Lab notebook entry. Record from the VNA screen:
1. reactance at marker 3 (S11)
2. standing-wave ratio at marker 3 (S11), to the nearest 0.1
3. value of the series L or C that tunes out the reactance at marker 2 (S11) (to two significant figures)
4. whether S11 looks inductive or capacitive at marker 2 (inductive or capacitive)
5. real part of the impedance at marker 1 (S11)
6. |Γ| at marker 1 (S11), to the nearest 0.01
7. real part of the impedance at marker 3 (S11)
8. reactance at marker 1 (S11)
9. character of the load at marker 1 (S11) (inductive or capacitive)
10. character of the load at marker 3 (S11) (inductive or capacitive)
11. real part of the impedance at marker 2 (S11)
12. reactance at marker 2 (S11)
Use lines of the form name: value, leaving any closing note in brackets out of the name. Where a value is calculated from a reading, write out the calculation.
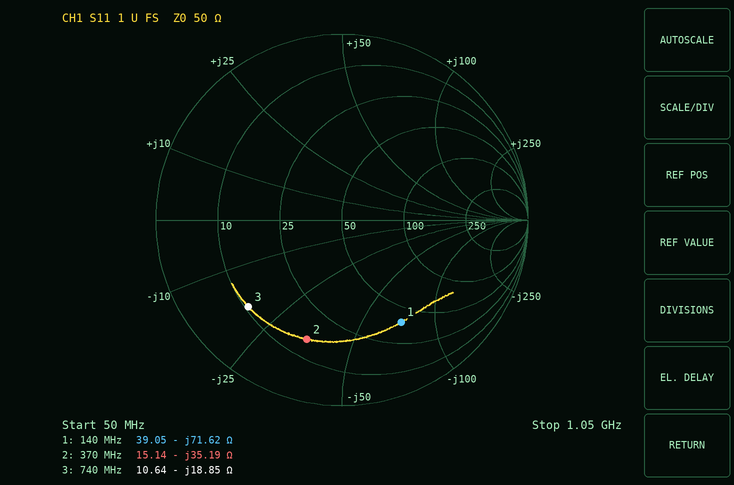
reactance at marker 3: -18.85 Ω
standing-wave ratio at marker 3 (S11), to the nearest 0.1: 5.4
value of the series L or C that tunes out the reactance at marker 2 (S11): L = 35.19 Ω/(2π × 370 MHz) ≈ 15 nH
whether S11 looks inductive or capacitive at marker 2: capacitive
real part of the impedance at marker 1: 39.05 Ω
|Γ| at marker 1 (S11), to the nearest 0.01: 0.63
real part of the impedance at marker 3: 10.64 Ω
reactance at marker 1: -71.62 Ω
character of the load at marker 1 (S11): capacitive
character of the load at marker 3 (S11): capacitive
real part of the impedance at marker 2: 15.14 Ω
reactance at marker 2: -35.19 Ω
